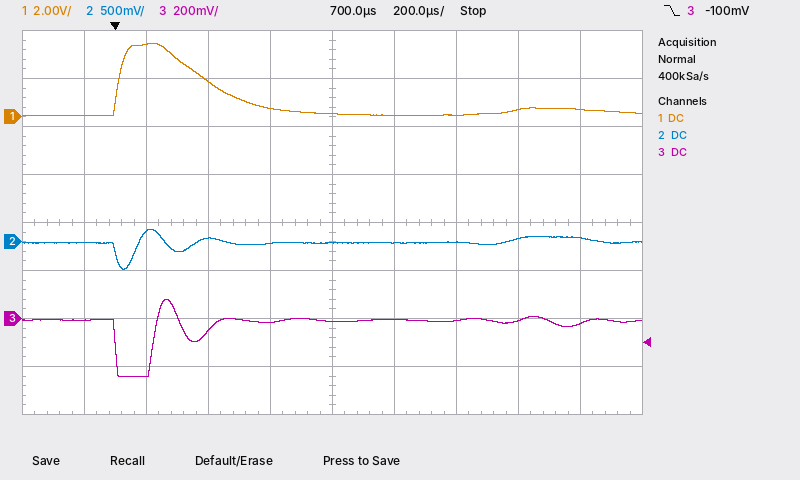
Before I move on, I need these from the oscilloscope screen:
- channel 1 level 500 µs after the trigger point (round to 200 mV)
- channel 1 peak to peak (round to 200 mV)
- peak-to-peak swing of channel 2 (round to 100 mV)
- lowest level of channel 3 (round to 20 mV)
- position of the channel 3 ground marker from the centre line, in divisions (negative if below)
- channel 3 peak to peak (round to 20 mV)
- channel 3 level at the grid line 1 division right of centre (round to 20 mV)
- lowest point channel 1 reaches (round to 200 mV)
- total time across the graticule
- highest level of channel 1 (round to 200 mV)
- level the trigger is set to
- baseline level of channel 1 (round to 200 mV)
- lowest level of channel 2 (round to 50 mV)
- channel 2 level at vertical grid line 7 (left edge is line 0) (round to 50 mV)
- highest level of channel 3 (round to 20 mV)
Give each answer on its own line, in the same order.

400 mV
3.0 V
400 mV
-240 mV
-2.0 div
320 mV
0 mV
0.0 V
2 ms
3.0 V
-100 mV
200 mV
-300 mV
0 mV
80 mV
